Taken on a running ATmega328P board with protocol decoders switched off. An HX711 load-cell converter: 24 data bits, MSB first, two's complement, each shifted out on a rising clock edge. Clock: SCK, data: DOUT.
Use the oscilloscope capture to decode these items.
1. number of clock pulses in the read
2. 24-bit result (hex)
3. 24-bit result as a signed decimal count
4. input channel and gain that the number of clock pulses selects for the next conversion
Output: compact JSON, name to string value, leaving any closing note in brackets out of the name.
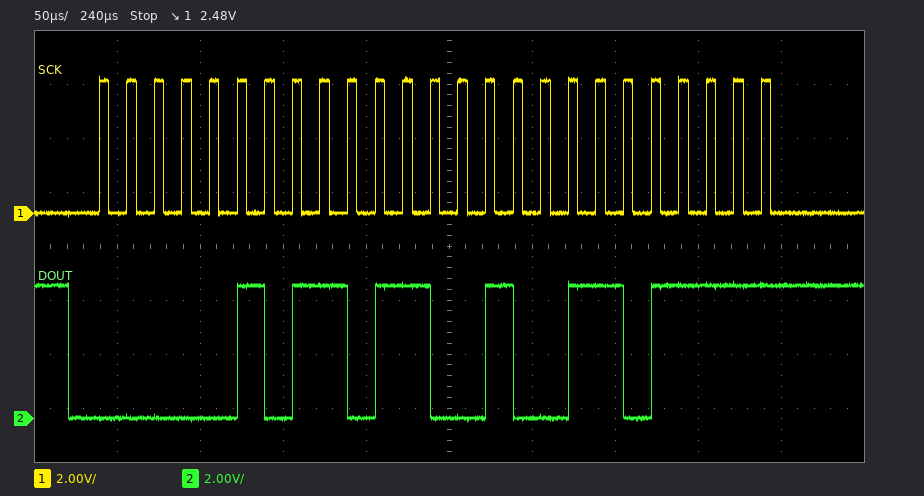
{"number of clock pulses in the read": "25", "24-bit result": "0x05B26F", "24-bit result as a signed decimal count": "373359", "input channel and gain that the number of clock pulses selects for the next conversion": "channel A, gain 128"}
